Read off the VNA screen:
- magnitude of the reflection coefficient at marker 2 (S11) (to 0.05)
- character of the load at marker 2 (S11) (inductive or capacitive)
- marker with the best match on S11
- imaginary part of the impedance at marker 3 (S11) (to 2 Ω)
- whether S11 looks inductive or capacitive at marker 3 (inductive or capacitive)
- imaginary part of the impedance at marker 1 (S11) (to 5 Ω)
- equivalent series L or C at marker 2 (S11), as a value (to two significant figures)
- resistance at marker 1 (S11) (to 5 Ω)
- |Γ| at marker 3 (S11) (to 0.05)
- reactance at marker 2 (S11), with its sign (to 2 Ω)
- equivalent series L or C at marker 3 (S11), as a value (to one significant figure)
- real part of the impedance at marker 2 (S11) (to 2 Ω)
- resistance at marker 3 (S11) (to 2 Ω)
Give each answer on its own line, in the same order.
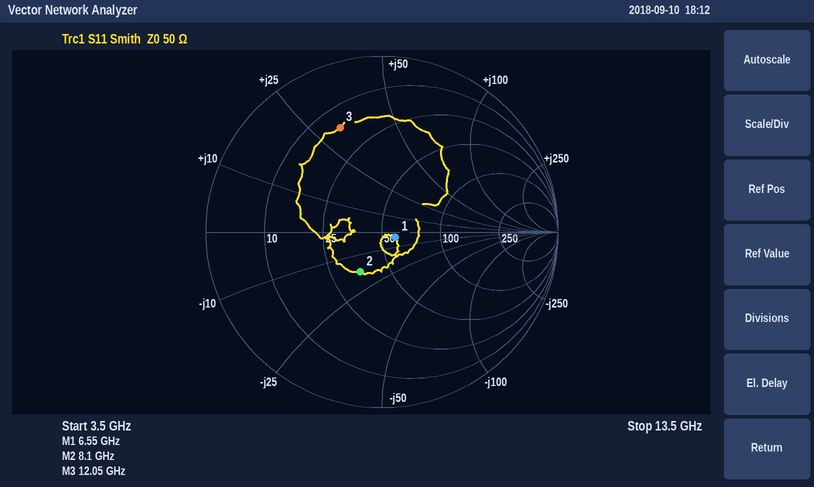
0.25
capacitive
marker 1
+32 Ω
inductive
-5 Ω
1.1 pF
60 Ω
0.65
-18 Ω
400 pH
36 Ω
16 Ω
